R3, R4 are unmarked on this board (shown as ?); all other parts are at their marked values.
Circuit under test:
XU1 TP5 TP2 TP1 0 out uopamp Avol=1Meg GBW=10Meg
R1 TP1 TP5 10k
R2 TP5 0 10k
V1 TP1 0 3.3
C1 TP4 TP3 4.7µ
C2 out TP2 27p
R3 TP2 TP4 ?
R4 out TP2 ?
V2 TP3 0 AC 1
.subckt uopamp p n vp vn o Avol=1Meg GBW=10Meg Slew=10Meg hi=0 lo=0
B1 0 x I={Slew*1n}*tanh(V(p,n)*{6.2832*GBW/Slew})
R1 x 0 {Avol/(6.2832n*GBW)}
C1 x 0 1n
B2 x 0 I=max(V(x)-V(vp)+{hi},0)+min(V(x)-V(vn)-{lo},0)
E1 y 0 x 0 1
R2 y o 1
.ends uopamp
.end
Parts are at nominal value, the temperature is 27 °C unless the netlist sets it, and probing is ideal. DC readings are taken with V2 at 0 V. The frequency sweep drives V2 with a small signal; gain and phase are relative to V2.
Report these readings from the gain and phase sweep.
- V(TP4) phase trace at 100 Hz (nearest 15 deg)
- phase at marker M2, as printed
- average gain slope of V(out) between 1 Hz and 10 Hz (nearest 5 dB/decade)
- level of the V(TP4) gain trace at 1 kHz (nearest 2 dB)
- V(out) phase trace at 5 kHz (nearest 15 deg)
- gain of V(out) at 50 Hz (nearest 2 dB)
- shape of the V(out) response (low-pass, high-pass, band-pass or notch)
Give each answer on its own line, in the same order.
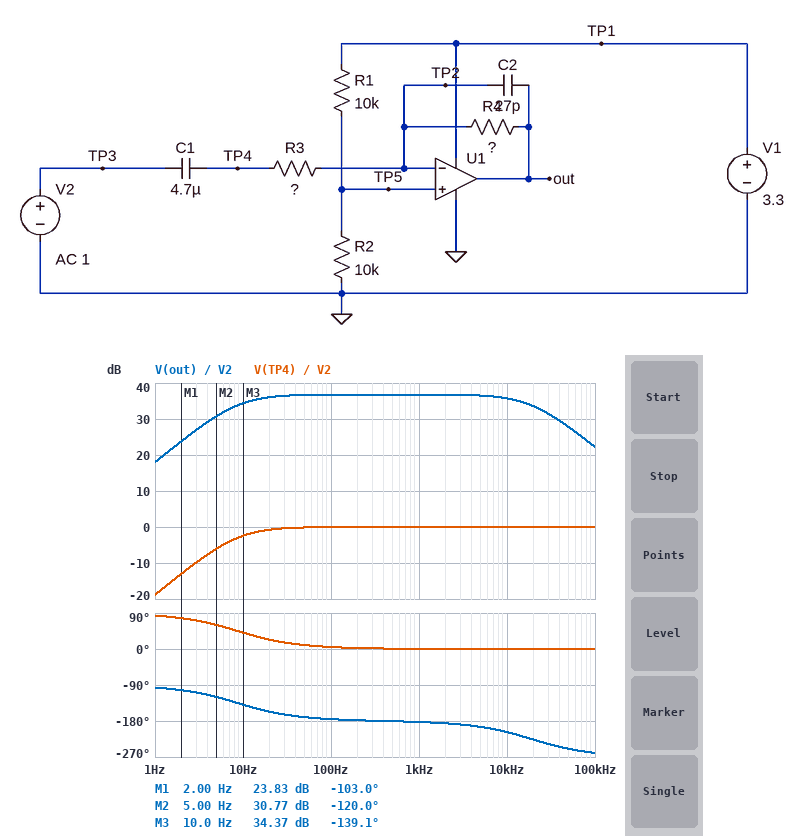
0 deg
-120.0 deg
15 dB/decade
0 dB
-195 deg
36 dB
band-pass
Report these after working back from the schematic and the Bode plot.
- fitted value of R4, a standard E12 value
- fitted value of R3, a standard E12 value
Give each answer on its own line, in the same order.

270 kΩ
3.9 kΩ
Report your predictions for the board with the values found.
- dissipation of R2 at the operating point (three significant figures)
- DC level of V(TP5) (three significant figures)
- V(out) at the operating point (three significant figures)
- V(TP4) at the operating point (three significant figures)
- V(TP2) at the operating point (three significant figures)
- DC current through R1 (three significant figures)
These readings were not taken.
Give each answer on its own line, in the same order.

272 µW
1.65 V
1.65 V
1.65 V
1.65 V
165 µA
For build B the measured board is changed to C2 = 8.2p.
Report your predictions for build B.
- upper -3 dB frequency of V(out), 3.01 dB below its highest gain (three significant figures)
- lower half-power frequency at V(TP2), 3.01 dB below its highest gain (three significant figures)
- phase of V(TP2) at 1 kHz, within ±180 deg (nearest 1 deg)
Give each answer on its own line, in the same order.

47.9 kHz
47.6 kHz
89 deg
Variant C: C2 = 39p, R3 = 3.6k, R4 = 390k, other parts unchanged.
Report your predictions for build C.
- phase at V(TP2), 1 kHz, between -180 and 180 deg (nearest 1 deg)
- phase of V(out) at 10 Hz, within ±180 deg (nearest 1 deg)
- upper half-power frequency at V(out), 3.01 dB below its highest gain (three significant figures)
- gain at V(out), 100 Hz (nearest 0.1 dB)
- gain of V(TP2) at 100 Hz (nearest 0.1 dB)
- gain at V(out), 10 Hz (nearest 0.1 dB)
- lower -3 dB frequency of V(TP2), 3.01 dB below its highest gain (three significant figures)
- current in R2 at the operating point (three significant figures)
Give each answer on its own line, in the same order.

84 deg
-137 deg
9.42 kHz
40.7 dB
-59.3 dB
37.9 dB
9.38 kHz
165 µA
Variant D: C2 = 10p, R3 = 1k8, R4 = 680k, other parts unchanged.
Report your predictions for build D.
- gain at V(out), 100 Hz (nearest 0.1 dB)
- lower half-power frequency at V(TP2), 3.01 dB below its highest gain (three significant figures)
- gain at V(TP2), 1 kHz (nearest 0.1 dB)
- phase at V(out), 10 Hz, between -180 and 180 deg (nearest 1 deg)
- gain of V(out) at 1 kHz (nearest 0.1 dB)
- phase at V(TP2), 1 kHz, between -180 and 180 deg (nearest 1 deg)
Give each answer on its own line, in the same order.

51.4 dB
12.4 kHz
-28.5 dB
-118 deg
51.5 dB
86 deg
